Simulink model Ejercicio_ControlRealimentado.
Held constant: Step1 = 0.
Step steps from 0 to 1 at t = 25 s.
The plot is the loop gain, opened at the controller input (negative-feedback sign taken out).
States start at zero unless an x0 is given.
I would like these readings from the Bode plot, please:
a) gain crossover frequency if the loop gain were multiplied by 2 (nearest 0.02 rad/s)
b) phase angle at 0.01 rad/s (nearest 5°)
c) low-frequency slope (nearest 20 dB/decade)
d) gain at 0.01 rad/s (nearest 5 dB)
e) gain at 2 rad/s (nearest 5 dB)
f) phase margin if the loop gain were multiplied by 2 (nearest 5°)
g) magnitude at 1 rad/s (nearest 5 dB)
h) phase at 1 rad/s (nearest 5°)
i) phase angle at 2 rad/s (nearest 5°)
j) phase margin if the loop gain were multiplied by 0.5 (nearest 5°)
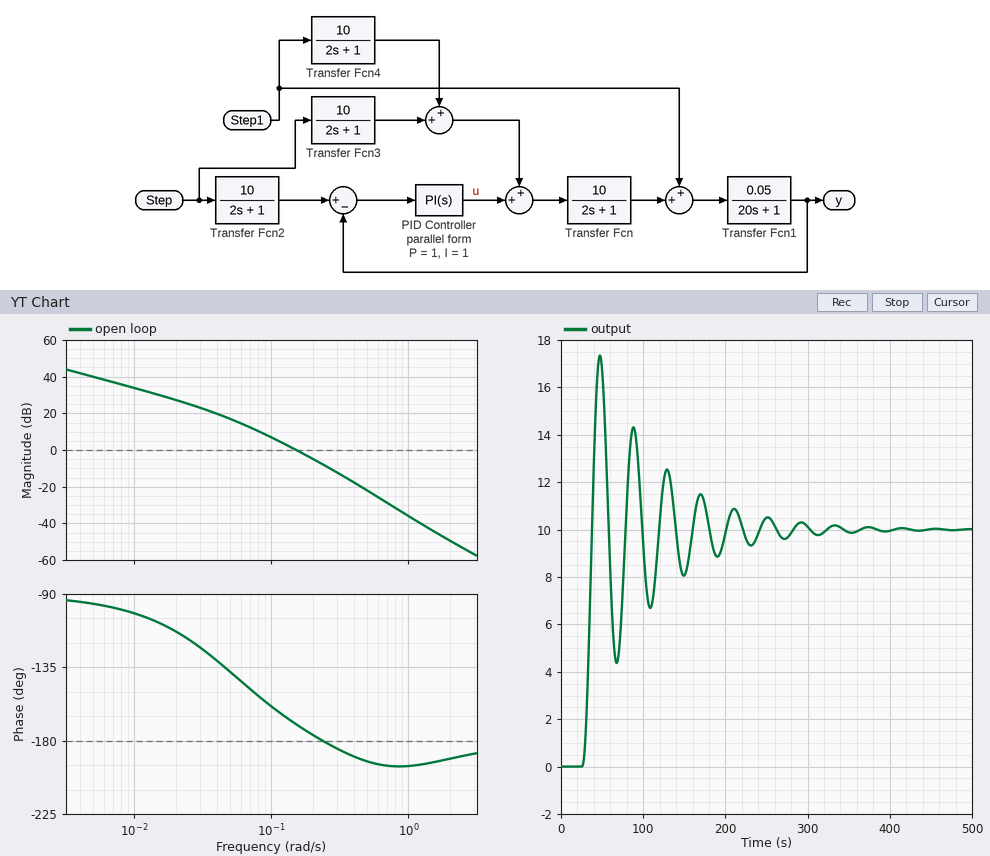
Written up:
0.22 rad/s
-100°
-20 dB/decade
35 dB
-50 dB
0°
-35 dB
-195°
-190°
20°
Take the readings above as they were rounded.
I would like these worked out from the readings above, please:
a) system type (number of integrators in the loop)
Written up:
1
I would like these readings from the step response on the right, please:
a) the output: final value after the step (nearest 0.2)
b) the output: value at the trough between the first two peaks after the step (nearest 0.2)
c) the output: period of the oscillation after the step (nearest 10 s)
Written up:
10.0
4.4
40 s
